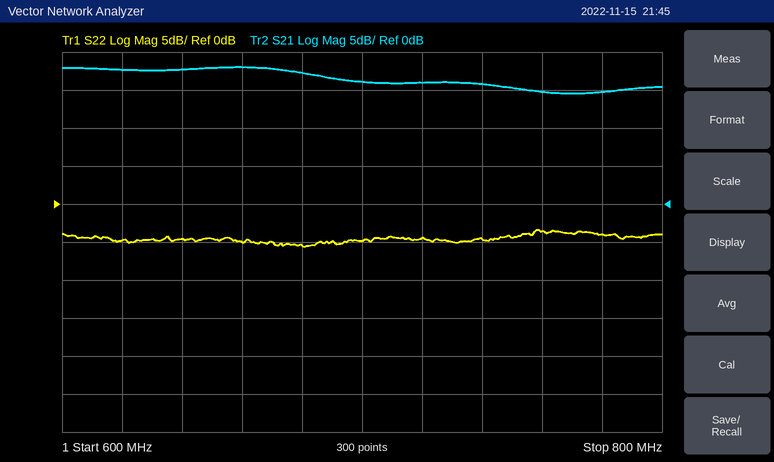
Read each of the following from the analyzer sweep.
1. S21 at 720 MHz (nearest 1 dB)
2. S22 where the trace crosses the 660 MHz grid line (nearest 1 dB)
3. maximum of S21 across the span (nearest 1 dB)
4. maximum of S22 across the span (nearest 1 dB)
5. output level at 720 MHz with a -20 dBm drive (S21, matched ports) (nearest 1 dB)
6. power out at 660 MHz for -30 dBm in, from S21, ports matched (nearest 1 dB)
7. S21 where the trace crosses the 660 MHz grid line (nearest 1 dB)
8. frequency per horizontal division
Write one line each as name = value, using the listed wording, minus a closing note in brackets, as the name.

S21 at 720 MHz = 16 dB
S22 where the trace crosses the 660 MHz grid line = -5 dB
maximum of S21 across the span = 18 dB
maximum of S22 across the span = -3 dB
output level at 720 MHz with a -20 dBm drive (S21, matched ports) = -4 dBm
power out at 660 MHz for -30 dBm in, from S21, ports matched = -12 dBm
S21 where the trace crosses the 660 MHz grid line = 18 dB
frequency per horizontal division = 20 MHz
